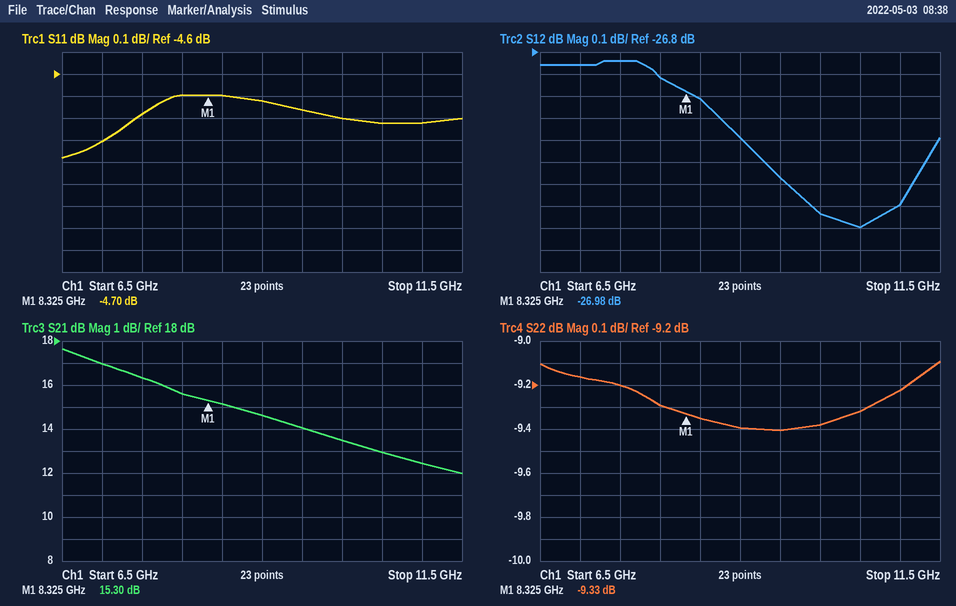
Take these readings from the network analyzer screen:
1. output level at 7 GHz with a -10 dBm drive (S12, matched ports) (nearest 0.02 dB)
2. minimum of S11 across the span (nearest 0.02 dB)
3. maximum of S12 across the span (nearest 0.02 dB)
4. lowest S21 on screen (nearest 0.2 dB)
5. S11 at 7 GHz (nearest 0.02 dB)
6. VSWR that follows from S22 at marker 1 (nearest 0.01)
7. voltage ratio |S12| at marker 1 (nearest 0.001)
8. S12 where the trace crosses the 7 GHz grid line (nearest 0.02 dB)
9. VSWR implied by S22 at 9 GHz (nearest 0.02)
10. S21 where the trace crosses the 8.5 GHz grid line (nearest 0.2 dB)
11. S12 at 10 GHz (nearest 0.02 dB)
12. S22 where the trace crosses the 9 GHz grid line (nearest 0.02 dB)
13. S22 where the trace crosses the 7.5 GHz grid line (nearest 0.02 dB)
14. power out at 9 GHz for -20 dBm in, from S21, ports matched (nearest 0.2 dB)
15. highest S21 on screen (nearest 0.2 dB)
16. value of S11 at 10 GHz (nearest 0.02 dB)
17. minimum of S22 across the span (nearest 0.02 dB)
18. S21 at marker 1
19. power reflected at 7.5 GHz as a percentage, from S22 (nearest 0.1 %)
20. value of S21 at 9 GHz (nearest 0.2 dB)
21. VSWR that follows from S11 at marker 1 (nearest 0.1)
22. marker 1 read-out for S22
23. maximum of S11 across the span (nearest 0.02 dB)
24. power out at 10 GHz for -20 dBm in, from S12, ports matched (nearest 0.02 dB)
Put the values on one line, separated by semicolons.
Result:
-36.86 dBm; -4.98 dB; -26.84 dB; 12.0 dB; -4.90 dB; 2.04; 0.045; -26.86 dB; 2.02; 15.2 dB; -27.54 dB; -9.40 dB; -9.20 dB; -5.4 dBm; 17.6 dB; -4.80 dB; -9.40 dB; 15.30 dB; 12.0 %; 14.6 dB; 3.8; -9.33 dB; -4.70 dB; -47.54 dBm
